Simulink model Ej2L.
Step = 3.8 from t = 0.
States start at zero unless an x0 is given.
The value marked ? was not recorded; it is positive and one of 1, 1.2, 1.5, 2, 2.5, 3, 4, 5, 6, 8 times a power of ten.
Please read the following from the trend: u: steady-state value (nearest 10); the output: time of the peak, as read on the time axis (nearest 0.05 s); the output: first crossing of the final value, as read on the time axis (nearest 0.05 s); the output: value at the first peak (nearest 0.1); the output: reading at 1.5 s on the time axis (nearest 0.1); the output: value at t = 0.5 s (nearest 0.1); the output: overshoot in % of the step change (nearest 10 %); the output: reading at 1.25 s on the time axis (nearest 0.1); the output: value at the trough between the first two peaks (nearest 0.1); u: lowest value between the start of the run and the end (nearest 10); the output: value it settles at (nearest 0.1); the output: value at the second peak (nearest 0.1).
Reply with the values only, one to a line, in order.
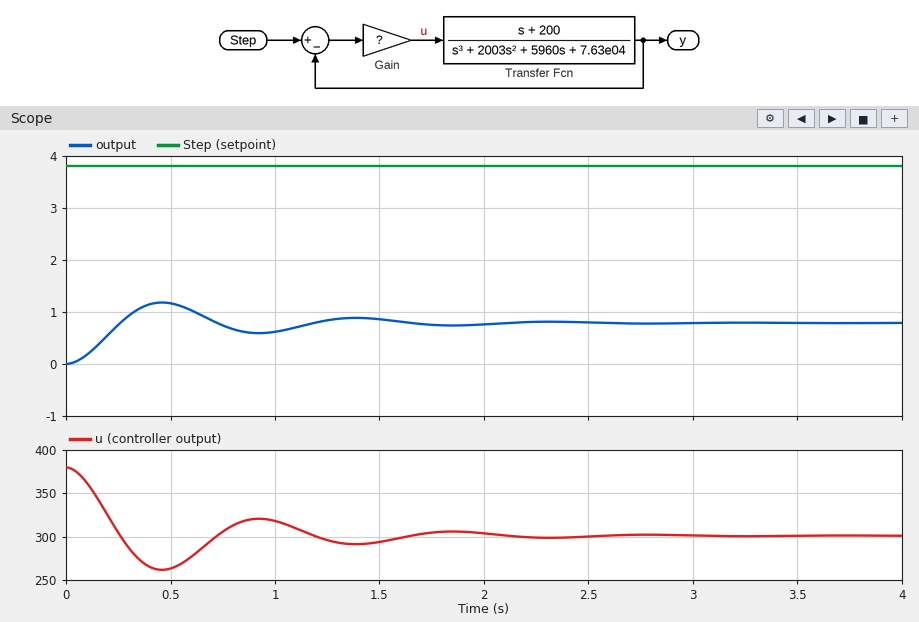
300
0.45 s
0.25 s
1.2
0.9
1.2
50 %
0.8
0.6
260
0.8
0.9
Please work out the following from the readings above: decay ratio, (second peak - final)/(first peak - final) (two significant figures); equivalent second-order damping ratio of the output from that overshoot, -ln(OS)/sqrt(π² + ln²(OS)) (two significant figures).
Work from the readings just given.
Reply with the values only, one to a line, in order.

0.25
0.22
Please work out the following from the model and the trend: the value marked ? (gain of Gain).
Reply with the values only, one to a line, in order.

100
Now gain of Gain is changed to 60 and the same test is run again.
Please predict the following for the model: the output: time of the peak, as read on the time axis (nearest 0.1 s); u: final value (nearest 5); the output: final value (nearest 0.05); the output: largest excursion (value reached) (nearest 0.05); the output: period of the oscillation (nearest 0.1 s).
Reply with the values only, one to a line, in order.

0.5 s
195
0.50
0.75
1.0 s
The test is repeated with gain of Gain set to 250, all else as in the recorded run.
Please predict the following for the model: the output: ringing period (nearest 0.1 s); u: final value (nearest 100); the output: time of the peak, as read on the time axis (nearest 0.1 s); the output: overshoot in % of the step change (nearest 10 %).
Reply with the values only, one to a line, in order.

0.8 s
600
0.4 s
50 %
